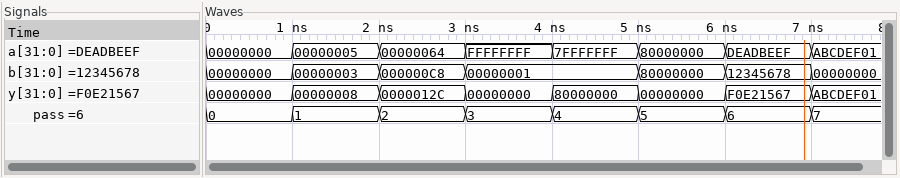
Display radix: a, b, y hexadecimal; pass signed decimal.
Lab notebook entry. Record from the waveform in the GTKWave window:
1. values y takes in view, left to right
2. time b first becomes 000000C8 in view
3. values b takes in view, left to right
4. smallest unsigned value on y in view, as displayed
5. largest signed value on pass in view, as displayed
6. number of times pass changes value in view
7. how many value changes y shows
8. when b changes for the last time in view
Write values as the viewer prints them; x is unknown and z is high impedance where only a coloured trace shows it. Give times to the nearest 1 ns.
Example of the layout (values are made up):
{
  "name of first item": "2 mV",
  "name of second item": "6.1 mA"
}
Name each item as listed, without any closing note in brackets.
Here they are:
{
  "values y takes in view, left to right": "00000000, 00000008, 0000012C, 00000000, 80000000, 00000000, F0E21567, ABCDEF01",
  "time b first becomes 000000C8 in view": "2 ns",
  "values b takes in view, left to right": "00000000, 00000003, 000000C8, 00000001, 80000000, 12345678, 00000000",
  "smallest unsigned value on y in view, as displayed": "00000000",
  "largest signed value on pass in view, as displayed": "7",
  "number of times pass changes value in view": "7",
  "how many value changes y shows": "7",
  "when b changes for the last time in view": "7 ns"
}
